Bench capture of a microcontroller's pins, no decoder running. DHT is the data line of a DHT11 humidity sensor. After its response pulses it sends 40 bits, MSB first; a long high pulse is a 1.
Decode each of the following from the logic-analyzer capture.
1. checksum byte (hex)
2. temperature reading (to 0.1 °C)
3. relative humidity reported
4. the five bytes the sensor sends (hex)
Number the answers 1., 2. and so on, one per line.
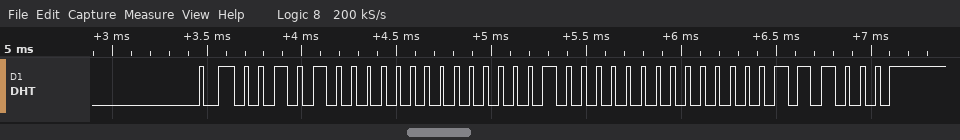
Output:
1. 0x38
2. 16.0 °C
3. 40 %
4. 28 00 10 00 38
